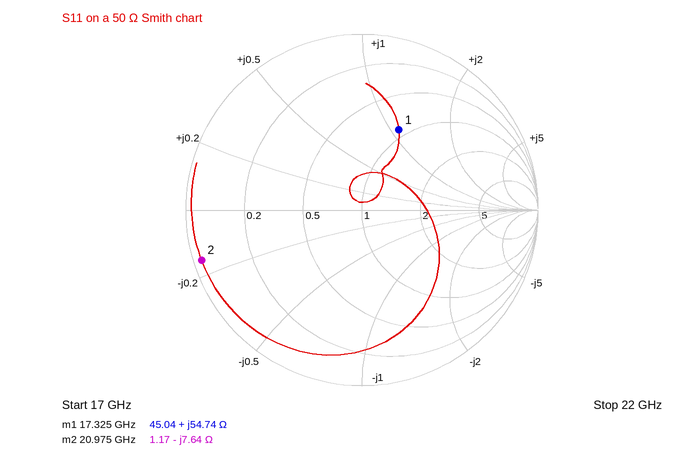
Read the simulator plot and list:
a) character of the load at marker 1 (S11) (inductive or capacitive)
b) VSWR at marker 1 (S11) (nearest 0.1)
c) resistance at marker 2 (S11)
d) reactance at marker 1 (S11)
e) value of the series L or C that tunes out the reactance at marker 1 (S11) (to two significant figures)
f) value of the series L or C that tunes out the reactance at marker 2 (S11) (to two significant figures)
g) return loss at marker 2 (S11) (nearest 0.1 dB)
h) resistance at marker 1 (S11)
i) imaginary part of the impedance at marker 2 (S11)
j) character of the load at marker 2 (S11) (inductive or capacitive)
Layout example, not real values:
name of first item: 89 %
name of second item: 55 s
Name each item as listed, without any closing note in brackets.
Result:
character of the load at marker 1 (S11): inductive
VSWR at marker 1 (S11): 3.0
resistance at marker 2: 1.17 Ω
reactance at marker 1: +54.74 Ω
value of the series L or C that tunes out the reactance at marker 1 (S11): 170 fF
value of the series L or C that tunes out the reactance at marker 2 (S11): 58 pH
return loss at marker 2 (S11): 0.4 dB
resistance at marker 1: 45.04 Ω
imaginary part of the impedance at marker 2: -7.64 Ω
character of the load at marker 2 (S11): capacitive
